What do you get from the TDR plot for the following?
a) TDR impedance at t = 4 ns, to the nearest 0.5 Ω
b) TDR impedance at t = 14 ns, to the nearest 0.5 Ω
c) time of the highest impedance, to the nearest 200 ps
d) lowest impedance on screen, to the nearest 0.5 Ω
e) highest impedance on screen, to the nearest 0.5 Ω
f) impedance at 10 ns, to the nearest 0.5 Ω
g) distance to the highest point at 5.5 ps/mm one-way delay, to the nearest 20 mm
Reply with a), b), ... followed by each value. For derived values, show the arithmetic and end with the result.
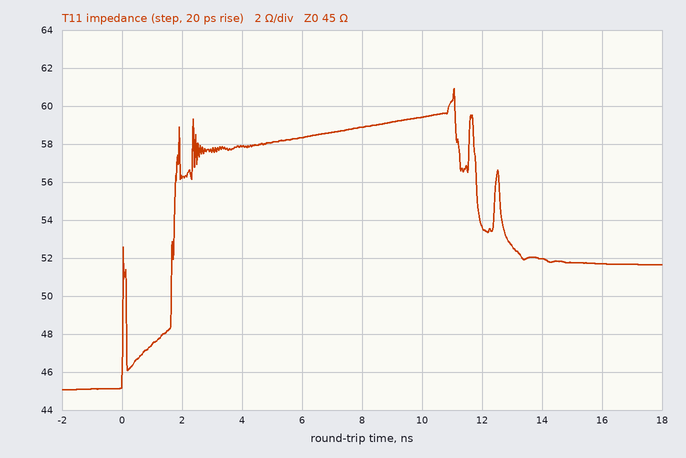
a) 58.0 Ω
b) 52.0 Ω
c) 11.0 ns
d) 45.0 Ω
e) 61.0 Ω
f) 59.5 Ω
g) 11.0 ns / 2 / 5.5 ps/mm ≈ 1.00 m
